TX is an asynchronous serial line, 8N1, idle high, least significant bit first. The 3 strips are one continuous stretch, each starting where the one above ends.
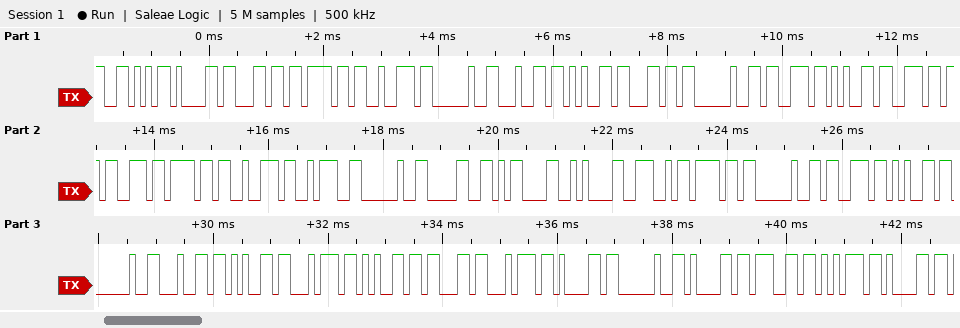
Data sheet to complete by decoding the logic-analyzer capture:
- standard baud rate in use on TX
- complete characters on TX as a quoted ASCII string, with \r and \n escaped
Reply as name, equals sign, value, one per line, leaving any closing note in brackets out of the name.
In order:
standard baud rate in use on TX = 9600 baud
complete characters on TX as a quoted ASCII string, with \r and \n escaped = "Valor del sensor: 0\r\nNo se detecta agua"
